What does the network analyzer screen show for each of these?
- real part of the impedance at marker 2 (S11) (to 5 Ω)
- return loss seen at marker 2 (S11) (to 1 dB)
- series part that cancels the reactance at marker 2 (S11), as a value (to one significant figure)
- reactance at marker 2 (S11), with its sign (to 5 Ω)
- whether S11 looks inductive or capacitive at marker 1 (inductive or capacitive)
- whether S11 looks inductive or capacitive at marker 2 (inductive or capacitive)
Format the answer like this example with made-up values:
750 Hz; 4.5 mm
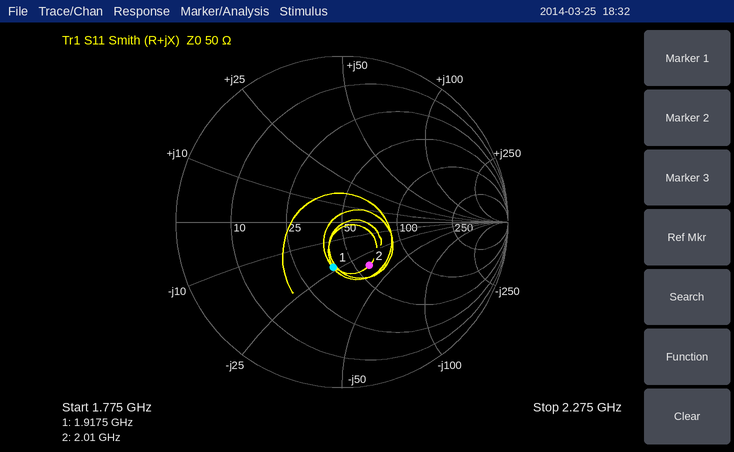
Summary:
60 Ω; 10 dB; 3 nH; -35 Ω; capacitive; capacitive
